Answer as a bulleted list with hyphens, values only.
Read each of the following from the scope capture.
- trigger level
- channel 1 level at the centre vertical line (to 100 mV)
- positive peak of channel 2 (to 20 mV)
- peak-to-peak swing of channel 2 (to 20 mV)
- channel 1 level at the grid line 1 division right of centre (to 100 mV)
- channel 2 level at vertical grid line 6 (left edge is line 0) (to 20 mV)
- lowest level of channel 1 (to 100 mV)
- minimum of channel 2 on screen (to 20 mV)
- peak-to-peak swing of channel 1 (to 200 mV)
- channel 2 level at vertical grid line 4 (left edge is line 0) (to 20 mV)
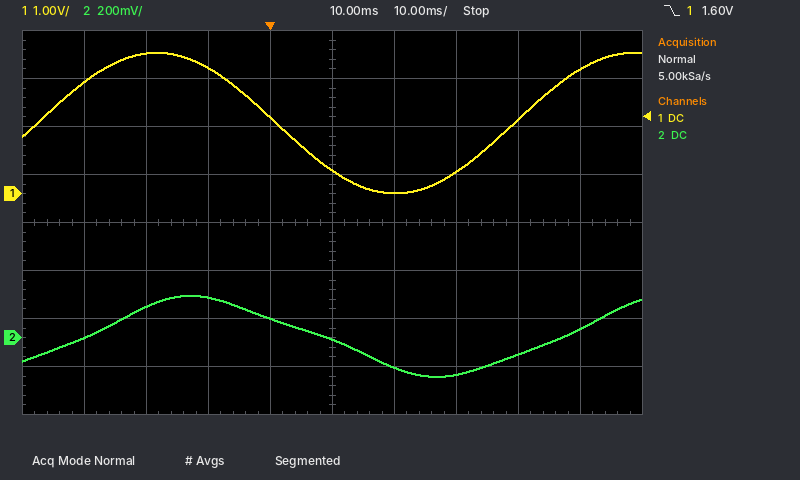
- 1.60 V
- 500 mV
- 180 mV
- 340 mV
- 0.0 V
- -120 mV
- 0.0 V
- -160 mV
- 3.0 V
- 80 mV
